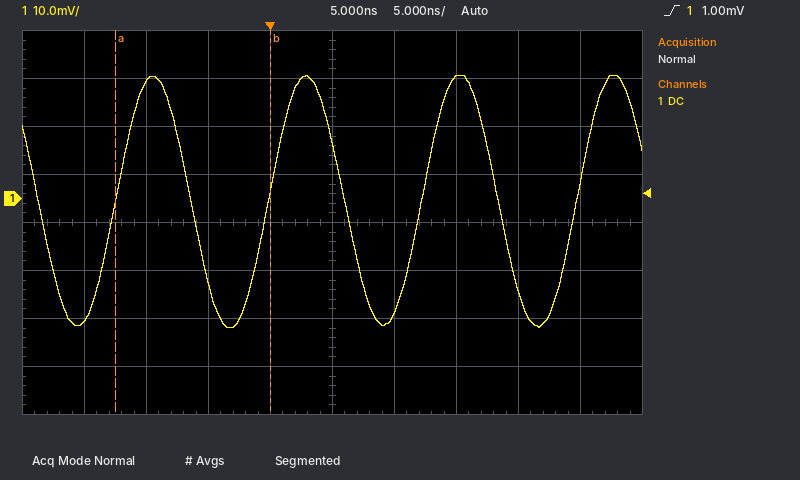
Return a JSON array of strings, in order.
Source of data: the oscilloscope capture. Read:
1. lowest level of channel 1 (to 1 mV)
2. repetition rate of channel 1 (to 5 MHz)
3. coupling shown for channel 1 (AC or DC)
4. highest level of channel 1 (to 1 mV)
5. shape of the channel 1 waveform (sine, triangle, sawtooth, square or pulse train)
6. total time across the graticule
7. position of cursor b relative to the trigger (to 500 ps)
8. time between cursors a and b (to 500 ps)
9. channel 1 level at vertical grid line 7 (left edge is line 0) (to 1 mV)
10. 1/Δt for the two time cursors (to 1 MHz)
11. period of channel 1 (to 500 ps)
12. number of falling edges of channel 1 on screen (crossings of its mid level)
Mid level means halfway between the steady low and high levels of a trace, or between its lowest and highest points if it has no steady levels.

["-27 mV", "80 MHz", "DC", "26 mV", "sine", "50 ns", "0.0 ns", "12.5 ns", "25 mV", "80 MHz", "12.5 ns", "4"]
